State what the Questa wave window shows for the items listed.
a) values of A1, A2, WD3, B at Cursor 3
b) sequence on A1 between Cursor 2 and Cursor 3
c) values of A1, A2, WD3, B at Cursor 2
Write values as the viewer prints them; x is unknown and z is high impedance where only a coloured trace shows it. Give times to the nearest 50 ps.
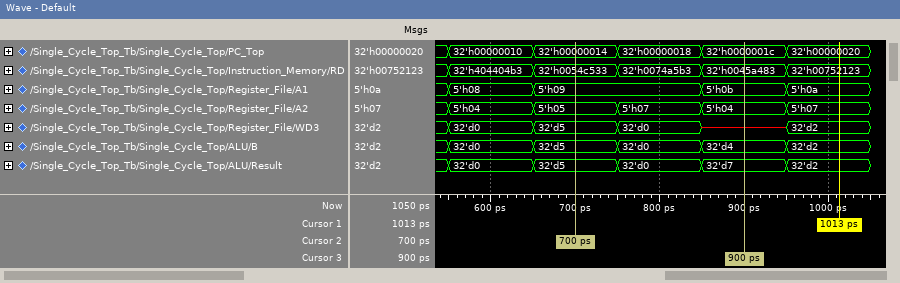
A1=5'h0b, A2=5'h04, WD3=x, B=32'd4
5'h09, 5'h0b
A1=5'h09, A2=5'h05, WD3=32'd5, B=32'd5
